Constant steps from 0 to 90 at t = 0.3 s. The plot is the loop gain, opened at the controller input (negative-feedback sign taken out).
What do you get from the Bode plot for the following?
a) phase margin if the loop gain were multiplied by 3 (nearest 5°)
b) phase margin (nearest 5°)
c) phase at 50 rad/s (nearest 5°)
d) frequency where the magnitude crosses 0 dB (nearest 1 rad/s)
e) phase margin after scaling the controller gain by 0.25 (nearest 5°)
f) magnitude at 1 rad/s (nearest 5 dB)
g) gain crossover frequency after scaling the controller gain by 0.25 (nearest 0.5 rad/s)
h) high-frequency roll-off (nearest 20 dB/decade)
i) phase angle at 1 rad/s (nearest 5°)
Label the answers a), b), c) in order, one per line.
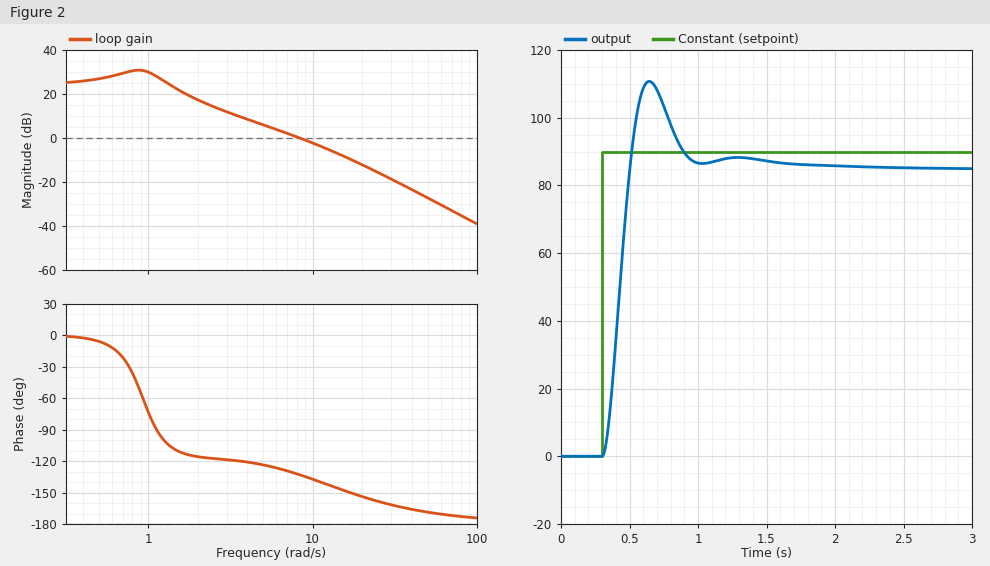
a) 30°
b) 45°
c) -170°
d) 8 rad/s
e) 60°
f) 30 dB
g) 3.0 rad/s
h) -40 dB/decade
i) -75°
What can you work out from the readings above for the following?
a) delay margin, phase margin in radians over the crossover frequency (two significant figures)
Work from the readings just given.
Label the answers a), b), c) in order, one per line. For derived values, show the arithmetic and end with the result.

a) 45 × π / 180 / 8 = 0.098 s
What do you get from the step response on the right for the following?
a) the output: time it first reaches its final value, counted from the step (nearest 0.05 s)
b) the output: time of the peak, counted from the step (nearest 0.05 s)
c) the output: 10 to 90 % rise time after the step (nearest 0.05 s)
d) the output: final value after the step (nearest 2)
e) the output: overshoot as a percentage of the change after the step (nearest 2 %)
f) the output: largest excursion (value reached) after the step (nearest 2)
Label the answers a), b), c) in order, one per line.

a) 0.20 s
b) 0.35 s
c) 0.15 s
d) 84
e) 30 %
f) 110
